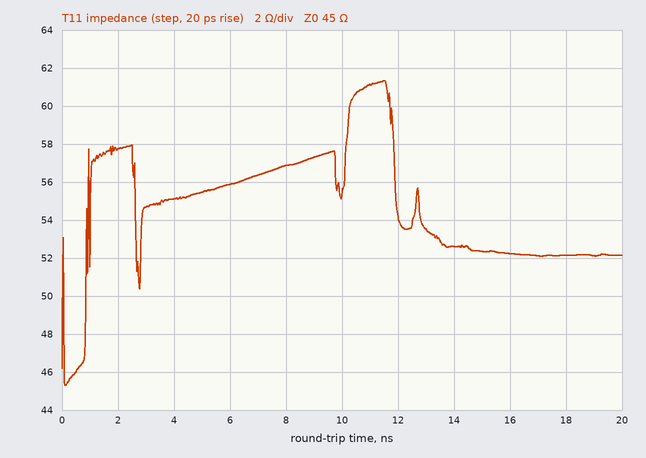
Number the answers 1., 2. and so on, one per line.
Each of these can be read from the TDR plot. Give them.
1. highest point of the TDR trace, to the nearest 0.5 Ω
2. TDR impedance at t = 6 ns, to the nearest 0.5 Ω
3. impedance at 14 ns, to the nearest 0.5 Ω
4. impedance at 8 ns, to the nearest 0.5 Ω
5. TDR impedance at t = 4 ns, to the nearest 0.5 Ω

1. 61.5 Ω
2. 56.0 Ω
3. 52.5 Ω
4. 57.0 Ω
5. 55.0 Ω
